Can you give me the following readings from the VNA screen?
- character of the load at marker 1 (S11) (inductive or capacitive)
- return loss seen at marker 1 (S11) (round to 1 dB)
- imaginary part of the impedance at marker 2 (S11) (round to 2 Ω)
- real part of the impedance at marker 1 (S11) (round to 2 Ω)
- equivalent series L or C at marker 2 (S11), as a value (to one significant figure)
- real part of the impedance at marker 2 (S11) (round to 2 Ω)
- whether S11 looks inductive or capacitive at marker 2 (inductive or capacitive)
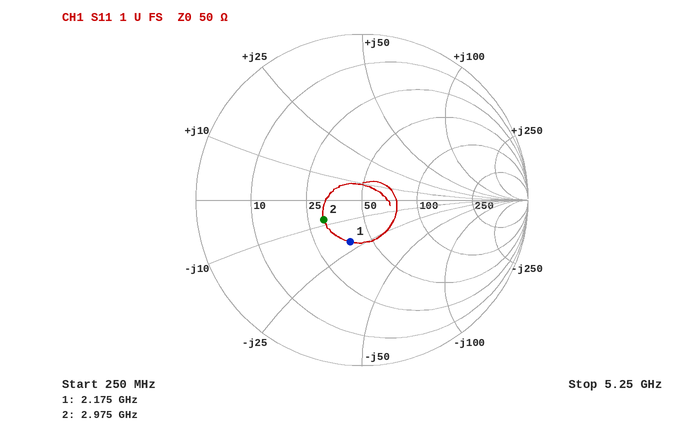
capacitive
12 dB
-8 Ω
38 Ω
7 pF
30 Ω
capacitive
